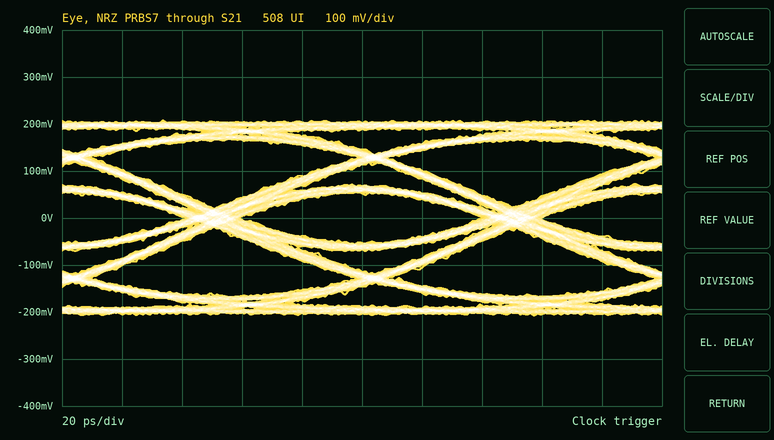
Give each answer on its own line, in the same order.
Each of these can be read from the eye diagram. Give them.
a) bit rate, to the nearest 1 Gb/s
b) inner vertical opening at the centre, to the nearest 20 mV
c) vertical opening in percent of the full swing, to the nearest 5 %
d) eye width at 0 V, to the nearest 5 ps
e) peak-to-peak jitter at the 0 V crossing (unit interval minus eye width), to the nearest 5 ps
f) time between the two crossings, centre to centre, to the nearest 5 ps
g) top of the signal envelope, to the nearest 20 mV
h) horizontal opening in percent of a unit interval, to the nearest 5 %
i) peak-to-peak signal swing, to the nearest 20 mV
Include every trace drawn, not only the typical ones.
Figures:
10 Gb/s
100 mV
25 %
80 ps
20 ps
100 ps
200 mV
80 %
420 mV
